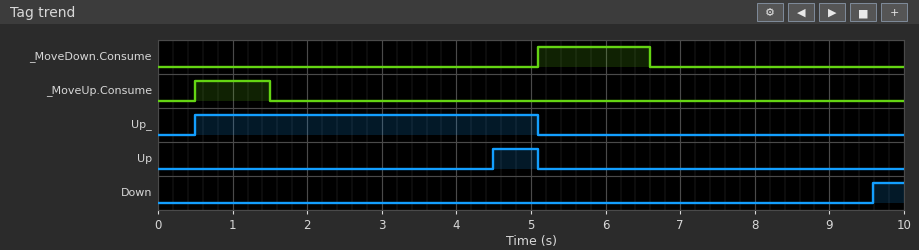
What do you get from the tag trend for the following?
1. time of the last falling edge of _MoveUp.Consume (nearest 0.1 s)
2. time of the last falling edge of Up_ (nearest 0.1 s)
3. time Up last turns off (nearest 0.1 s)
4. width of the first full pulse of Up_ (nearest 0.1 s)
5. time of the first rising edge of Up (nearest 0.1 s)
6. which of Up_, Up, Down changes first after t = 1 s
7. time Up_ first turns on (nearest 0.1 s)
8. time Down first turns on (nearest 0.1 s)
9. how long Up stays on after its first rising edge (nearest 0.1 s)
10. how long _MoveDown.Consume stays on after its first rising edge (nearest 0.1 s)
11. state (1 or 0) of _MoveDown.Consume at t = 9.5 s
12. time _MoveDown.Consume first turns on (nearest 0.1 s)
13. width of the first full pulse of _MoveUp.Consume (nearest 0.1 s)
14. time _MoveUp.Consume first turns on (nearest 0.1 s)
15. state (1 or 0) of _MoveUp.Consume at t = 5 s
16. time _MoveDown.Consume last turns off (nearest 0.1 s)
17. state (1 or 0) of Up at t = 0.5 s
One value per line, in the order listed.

1.5 s
5.1 s
5.1 s
4.6 s
4.5 s
Up
0.5 s
9.6 s
0.6 s
1.5 s
0
5.1 s
1.0 s
0.5 s
0
6.6 s
0
